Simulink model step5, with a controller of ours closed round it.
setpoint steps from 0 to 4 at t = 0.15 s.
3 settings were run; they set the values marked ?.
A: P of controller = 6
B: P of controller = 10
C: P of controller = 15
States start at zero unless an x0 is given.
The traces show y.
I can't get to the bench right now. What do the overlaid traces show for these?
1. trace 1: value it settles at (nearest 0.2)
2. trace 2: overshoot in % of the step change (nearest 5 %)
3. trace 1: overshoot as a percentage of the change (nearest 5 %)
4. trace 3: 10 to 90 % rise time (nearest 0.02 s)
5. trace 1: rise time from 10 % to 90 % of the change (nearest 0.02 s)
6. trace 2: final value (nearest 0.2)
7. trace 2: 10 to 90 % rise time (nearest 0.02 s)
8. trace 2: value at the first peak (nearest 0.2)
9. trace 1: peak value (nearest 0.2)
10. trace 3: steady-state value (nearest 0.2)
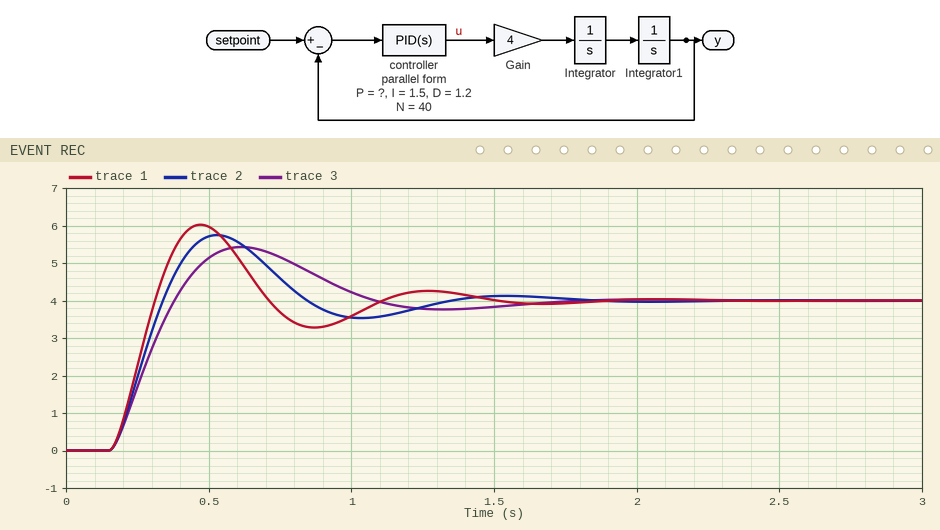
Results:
4.0
45 %
50 %
0.16 s
0.12 s
4.0
0.14 s
5.8
6.0
4.0
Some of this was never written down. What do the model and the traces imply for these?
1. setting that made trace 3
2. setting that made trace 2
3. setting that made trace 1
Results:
A
B
C
